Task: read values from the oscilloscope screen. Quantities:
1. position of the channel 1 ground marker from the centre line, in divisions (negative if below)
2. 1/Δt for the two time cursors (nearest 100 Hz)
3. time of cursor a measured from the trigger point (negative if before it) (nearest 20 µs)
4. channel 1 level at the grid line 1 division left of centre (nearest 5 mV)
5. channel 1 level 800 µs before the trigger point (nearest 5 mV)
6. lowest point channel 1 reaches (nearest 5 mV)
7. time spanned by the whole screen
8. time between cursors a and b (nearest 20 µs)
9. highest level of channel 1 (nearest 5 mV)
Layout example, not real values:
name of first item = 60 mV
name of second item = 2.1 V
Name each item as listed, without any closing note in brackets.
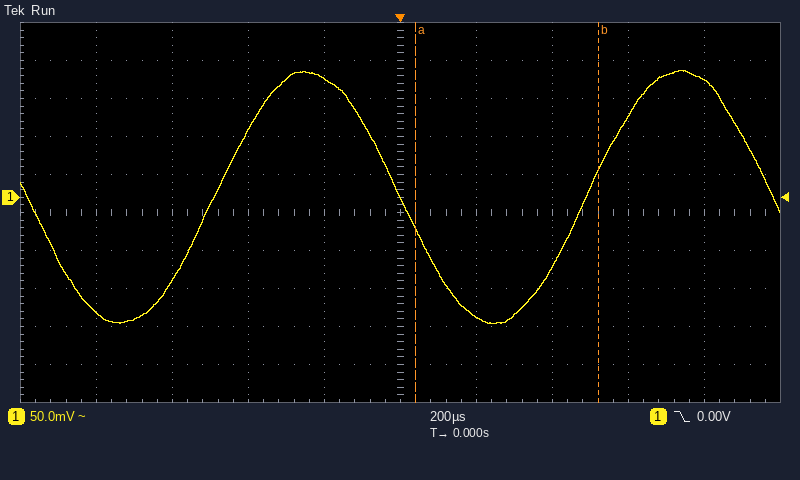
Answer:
position of the channel 1 ground marker from the centre line, in divisions = +0.4 div
1/Δt for the two time cursors = 2.1 kHz
time of cursor a measured from the trigger point (negative if before it) = +40 µs
channel 1 level at the grid line 1 division left of centre = 155 mV
channel 1 level 800 µs before the trigger point = -150 mV
lowest point channel 1 reaches = -165 mV
time spanned by the whole screen = 2 ms
time between cursors a and b = 480 µs
highest level of channel 1 = 165 mV
